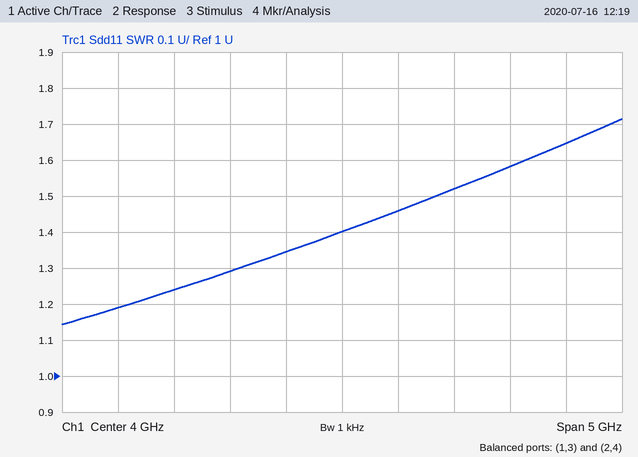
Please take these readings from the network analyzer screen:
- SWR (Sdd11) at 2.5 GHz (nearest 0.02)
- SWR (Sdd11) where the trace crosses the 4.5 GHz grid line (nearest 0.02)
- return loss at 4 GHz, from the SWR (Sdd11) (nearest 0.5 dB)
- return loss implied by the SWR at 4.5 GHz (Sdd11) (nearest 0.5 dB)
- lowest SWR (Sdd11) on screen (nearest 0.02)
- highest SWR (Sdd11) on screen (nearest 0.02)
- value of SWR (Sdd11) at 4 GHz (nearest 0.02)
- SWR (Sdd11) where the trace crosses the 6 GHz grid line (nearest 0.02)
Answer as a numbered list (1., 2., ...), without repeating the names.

1. 1.24
2. 1.46
3. 15.5 dB
4. 14.5 dB
5. 1.14
6. 1.72
7. 1.40
8. 1.64
